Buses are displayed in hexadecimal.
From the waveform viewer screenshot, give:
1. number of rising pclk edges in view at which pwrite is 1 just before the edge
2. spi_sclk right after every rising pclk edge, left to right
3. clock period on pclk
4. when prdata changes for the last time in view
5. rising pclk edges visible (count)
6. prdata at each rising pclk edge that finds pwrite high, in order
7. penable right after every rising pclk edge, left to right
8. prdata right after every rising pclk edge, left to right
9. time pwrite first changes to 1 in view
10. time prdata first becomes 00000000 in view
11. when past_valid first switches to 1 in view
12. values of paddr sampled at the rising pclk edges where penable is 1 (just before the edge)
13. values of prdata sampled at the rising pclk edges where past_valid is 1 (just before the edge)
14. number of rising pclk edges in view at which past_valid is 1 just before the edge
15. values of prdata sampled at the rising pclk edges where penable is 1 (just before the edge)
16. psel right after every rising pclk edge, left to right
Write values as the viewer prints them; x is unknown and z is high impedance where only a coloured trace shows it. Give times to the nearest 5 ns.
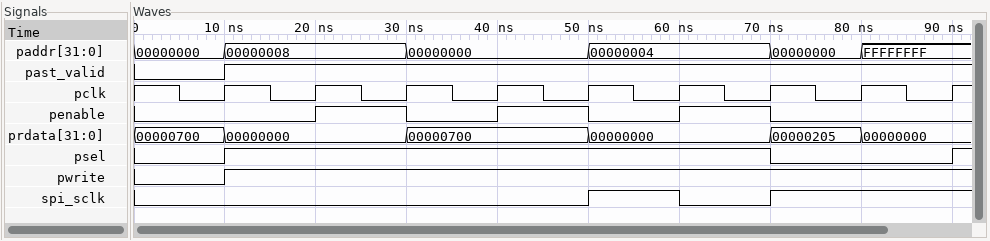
8
0 0 0 0 1 0 1 1 1
10 ns
80 ns
9
00000000, 00000000, 00000700, 00000700, 00000000, 00000000, 00000205, 00000000
0 1 0 1 0 1 0 0 0
00000000, 00000000, 00000700, 00000700, 00000000, 00000000, 00000205, 00000000, 00000000
10 ns
10 ns
10 ns
00000008, 00000000, 00000004
00000000, 00000000, 00000700, 00000700, 00000000, 00000000, 00000205, 00000000
8
00000000, 00000700, 00000000
1 1 1 1 1 1 0 0 1
